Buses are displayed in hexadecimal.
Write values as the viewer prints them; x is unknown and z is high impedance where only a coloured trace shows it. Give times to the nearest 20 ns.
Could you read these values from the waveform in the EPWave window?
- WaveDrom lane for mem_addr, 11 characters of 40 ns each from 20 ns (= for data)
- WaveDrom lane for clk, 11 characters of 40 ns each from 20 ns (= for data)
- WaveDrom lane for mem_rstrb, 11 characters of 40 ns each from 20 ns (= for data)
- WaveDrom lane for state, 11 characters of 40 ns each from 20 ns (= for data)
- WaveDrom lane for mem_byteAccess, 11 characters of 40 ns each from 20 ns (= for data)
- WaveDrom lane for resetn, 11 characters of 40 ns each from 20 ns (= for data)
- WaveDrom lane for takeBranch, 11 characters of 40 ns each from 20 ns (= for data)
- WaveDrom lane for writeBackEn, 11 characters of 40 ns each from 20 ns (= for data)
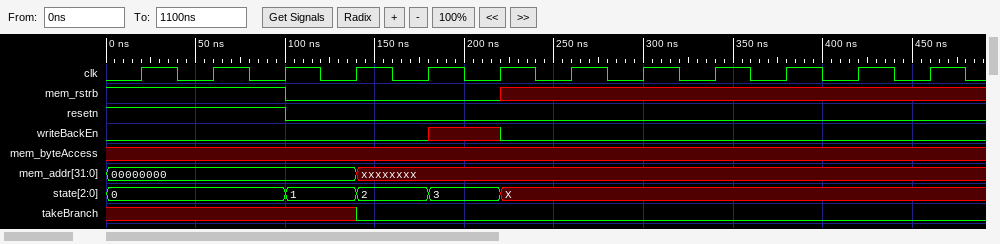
{name: 'mem_addr', wave: '=..x.......', data: '00000000'}
{name: 'clk', wave: 'p..........'}
{name: 'mem_rstrb', wave: '1.0..x.....'}
{name: 'state', wave: '=.====.....', data: '0 1 2 3 X'}
{name: 'mem_byteAccess', wave: 'x..........'}
{name: 'resetn', wave: '1.0........'}
{name: 'takeBranch', wave: 'x..0.......'}
{name: 'writeBackEn', wave: '0...x0.....'}
